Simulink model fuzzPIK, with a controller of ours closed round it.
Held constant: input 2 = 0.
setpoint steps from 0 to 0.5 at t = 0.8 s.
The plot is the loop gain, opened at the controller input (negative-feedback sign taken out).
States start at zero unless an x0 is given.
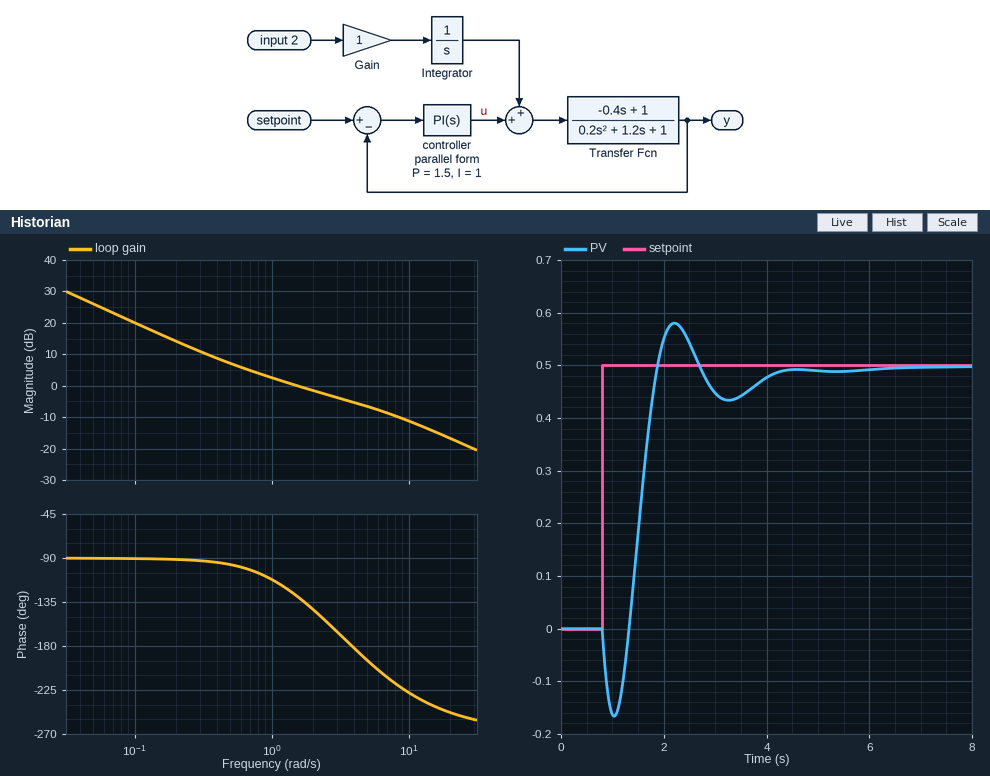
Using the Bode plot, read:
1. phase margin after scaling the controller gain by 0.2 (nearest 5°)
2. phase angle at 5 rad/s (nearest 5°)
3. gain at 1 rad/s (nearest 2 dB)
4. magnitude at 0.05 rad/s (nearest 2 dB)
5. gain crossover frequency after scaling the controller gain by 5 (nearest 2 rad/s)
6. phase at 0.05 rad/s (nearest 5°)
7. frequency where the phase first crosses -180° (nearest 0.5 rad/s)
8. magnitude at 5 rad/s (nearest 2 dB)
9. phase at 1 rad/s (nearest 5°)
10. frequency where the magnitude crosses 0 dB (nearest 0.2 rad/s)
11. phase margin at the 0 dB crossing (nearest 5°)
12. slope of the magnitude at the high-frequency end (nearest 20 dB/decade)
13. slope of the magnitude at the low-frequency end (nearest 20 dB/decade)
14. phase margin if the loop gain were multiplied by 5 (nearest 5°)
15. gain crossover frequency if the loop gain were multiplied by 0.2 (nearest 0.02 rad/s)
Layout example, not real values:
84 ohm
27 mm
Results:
90°
-195°
2 dB
26 dB
14 rad/s
-90°
4.0 rad/s
-6 dB
-110°
1.6 rad/s
50°
-20 dB/decade
-20 dB/decade
-60°
0.20 rad/s
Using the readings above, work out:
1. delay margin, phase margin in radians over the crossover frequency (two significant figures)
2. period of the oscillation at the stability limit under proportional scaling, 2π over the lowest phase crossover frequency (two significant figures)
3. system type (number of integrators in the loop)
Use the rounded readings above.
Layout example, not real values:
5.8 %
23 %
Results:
0.55 s
1.6 s
1
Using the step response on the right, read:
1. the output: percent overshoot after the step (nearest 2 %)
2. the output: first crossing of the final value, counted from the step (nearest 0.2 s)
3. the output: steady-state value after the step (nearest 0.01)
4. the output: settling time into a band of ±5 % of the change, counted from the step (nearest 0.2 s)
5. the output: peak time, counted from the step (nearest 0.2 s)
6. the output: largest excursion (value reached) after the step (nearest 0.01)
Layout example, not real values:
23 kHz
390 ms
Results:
16 %
1.0 s
0.50
3.2 s
1.4 s
0.58
